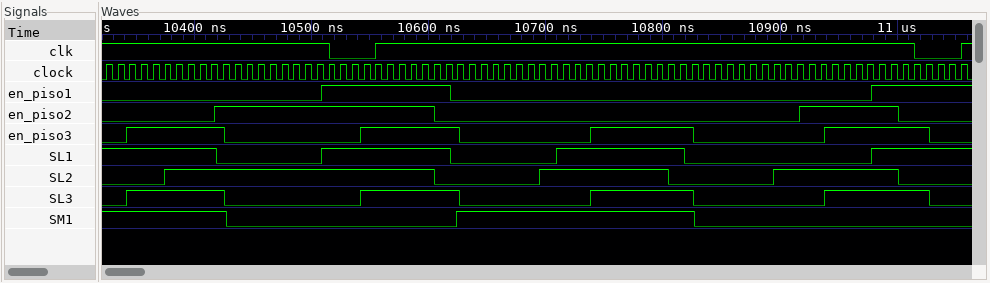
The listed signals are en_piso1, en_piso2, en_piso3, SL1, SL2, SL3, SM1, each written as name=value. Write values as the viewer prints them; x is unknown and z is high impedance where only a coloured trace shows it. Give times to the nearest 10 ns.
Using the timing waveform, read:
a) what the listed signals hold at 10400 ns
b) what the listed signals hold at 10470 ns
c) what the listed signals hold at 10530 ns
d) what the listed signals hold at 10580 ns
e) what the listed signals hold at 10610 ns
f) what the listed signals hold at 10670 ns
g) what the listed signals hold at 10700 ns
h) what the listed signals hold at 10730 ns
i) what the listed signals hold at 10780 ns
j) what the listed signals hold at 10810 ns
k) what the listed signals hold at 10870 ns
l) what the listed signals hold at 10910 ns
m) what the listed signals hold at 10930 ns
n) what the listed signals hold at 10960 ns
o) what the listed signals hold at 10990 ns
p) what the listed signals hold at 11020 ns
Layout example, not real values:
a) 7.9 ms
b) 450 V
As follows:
a) en_piso1=0, en_piso2=0, en_piso3=1, SL1=1, SL2=1, SL3=1, SM1=1
b) en_piso1=0, en_piso2=1, en_piso3=0, SL1=0, SL2=1, SL3=0, SM1=0
c) en_piso1=1, en_piso2=1, en_piso3=0, SL1=1, SL2=1, SL3=0, SM1=0
d) en_piso1=1, en_piso2=1, en_piso3=1, SL1=1, SL2=1, SL3=1, SM1=0
e) en_piso1=1, en_piso2=0, en_piso3=1, SL1=1, SL2=0, SL3=1, SM1=0
f) en_piso1=0, en_piso2=0, en_piso3=0, SL1=0, SL2=0, SL3=0, SM1=1
g) en_piso1=0, en_piso2=0, en_piso3=0, SL1=0, SL2=1, SL3=0, SM1=1
h) en_piso1=0, en_piso2=0, en_piso3=0, SL1=1, SL2=1, SL3=0, SM1=1
i) en_piso1=0, en_piso2=0, en_piso3=1, SL1=1, SL2=1, SL3=1, SM1=1
j) en_piso1=0, en_piso2=0, en_piso3=1, SL1=1, SL2=0, SL3=1, SM1=1
k) en_piso1=0, en_piso2=0, en_piso3=0, SL1=0, SL2=0, SL3=0, SM1=0
l) en_piso1=0, en_piso2=0, en_piso3=0, SL1=0, SL2=1, SL3=0, SM1=0
m) en_piso1=0, en_piso2=1, en_piso3=0, SL1=0, SL2=1, SL3=0, SM1=0
n) en_piso1=0, en_piso2=1, en_piso3=1, SL1=0, SL2=1, SL3=1, SM1=0
o) en_piso1=1, en_piso2=1, en_piso3=1, SL1=1, SL2=1, SL3=1, SM1=0
p) en_piso1=1, en_piso2=0, en_piso3=1, SL1=1, SL2=0, SL3=1, SM1=0
